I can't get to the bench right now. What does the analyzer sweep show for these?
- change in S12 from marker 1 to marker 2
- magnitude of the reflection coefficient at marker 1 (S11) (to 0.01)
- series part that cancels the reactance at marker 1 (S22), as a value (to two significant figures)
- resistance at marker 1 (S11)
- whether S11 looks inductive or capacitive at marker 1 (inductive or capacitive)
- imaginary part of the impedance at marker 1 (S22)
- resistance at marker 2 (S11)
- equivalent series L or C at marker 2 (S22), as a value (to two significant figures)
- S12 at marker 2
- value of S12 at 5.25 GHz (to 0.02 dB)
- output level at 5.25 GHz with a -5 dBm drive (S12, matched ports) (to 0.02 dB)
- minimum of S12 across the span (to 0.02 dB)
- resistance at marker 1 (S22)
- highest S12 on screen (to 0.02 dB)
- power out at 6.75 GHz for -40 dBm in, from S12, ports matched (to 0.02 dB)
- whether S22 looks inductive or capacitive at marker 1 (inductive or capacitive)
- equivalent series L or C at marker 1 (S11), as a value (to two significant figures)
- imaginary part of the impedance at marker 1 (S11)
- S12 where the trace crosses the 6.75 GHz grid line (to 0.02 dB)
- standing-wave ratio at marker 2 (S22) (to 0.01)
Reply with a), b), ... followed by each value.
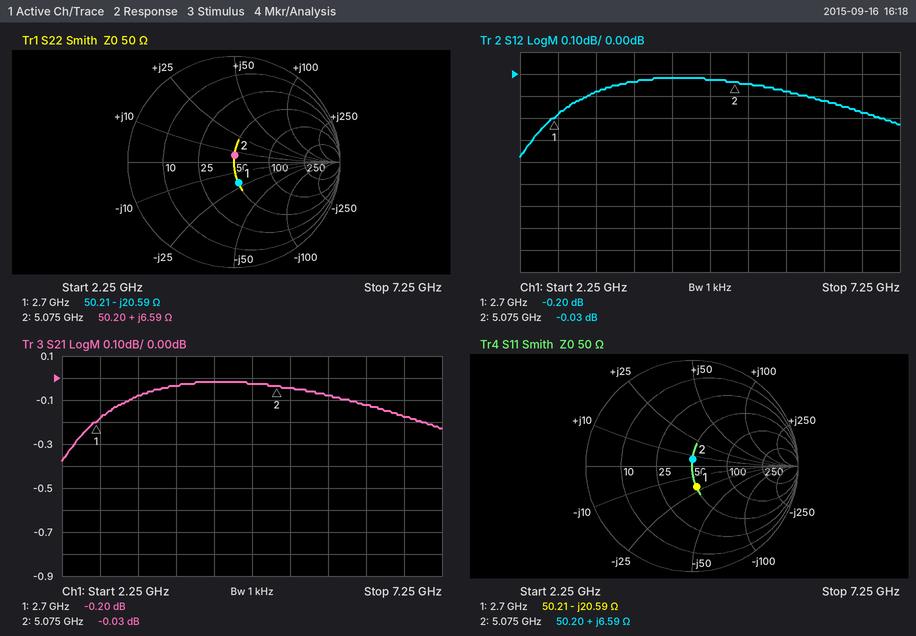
a) 0.17 dB
b) 0.20
c) 1.2 nH
d) 50.21 Ω
e) capacitive
f) -20.59 Ω
g) 50.20 Ω
h) 210 pH
i) -0.03 dB
j) -0.04 dB
k) -5.04 dBm
l) -0.38 dB
m) 50.21 Ω
n) -0.02 dB
o) -40.18 dBm
p) capacitive
q) 2.9 pF
r) -20.59 Ω
s) -0.18 dB
t) 1.14
